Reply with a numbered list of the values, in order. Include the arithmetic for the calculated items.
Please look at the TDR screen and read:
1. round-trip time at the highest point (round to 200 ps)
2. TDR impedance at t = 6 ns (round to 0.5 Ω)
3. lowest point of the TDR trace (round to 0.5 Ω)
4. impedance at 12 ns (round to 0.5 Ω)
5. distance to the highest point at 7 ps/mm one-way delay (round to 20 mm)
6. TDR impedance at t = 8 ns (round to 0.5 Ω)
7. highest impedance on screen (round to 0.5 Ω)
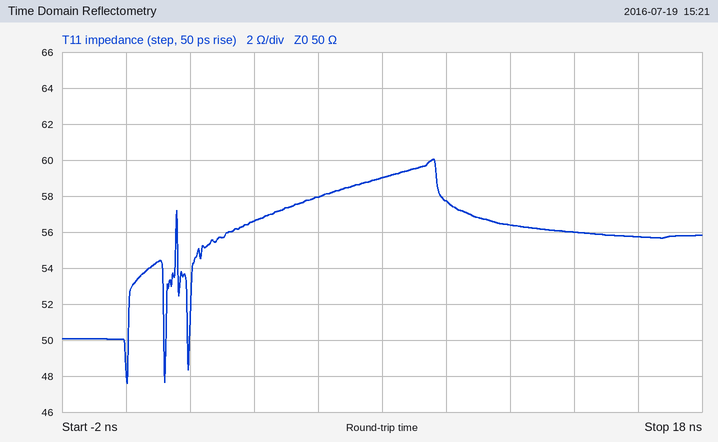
1. 9.6 ns
2. 58.0 Ω
3. 47.5 Ω
4. 56.5 Ω
5. 9.6 ns / 2 / 7 ps/mm ≈ 686 mm, so 680 mm to the nearest 20 mm
6. 59.0 Ω
7. 60.0 Ω
